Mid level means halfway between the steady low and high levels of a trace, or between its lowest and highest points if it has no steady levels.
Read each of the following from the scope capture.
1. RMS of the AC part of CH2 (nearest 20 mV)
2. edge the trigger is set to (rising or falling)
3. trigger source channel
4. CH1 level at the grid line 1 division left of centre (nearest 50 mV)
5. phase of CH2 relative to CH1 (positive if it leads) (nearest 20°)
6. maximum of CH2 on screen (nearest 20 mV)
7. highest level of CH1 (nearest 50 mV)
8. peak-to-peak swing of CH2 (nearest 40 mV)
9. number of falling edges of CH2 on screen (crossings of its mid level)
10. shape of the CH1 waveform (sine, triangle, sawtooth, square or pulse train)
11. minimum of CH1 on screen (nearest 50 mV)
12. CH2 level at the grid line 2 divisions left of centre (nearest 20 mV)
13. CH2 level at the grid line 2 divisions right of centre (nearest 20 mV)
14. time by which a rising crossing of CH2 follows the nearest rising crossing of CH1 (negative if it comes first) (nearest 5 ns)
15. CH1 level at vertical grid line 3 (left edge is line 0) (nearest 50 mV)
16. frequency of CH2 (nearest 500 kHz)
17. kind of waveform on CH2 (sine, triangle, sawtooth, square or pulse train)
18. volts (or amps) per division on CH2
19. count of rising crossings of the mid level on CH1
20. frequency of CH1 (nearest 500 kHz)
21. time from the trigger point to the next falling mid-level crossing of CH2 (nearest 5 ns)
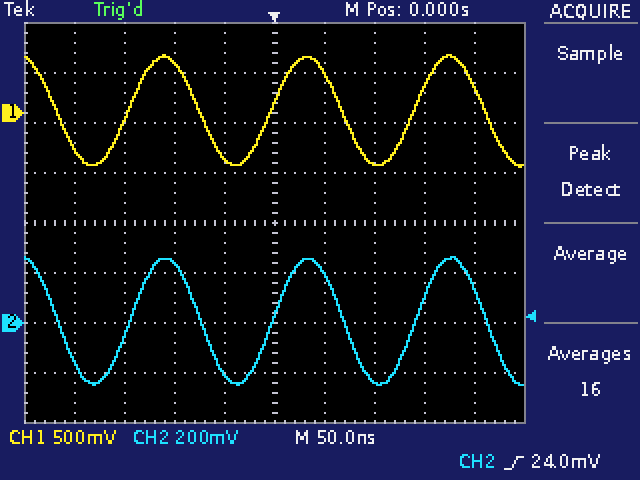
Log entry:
180 mV
rising
CH2
-450 mV
0°
260 mV
600 mV
520 mV
4
sine
-550 mV
240 mV
-240 mV
0 ns
500 mV
7.0 MHz
sine
200 mV
3
7.0 MHz
70 ns
